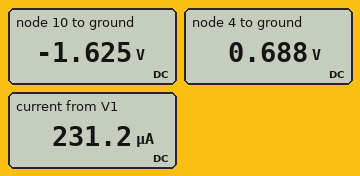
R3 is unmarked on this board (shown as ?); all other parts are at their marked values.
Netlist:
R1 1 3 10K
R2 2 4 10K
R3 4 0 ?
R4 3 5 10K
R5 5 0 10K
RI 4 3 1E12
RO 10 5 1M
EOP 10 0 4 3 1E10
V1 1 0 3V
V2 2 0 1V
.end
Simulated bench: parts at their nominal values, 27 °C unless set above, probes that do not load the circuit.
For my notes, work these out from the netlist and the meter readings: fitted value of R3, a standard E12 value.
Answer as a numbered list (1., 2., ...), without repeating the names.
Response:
1. 22 kΩ
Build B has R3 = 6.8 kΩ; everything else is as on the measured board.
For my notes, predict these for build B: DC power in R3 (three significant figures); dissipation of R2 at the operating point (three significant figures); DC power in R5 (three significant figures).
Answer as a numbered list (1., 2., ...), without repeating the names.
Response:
1. 24.1 µW
2. 35.4 µW
3. 480 µW
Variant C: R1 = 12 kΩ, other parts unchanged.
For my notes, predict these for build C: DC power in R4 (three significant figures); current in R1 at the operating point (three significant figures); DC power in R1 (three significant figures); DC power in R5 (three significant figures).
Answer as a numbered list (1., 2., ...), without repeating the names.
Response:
1. 371 µW
2. 193 µA
3. 446 µW
4. 154 µW
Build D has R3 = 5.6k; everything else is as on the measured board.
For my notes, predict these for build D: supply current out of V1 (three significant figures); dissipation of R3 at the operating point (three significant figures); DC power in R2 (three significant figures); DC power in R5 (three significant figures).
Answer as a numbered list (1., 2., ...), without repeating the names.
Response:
1. 264 µA
2. 23.0 µW
3. 41.1 µW
4. 521 µW
